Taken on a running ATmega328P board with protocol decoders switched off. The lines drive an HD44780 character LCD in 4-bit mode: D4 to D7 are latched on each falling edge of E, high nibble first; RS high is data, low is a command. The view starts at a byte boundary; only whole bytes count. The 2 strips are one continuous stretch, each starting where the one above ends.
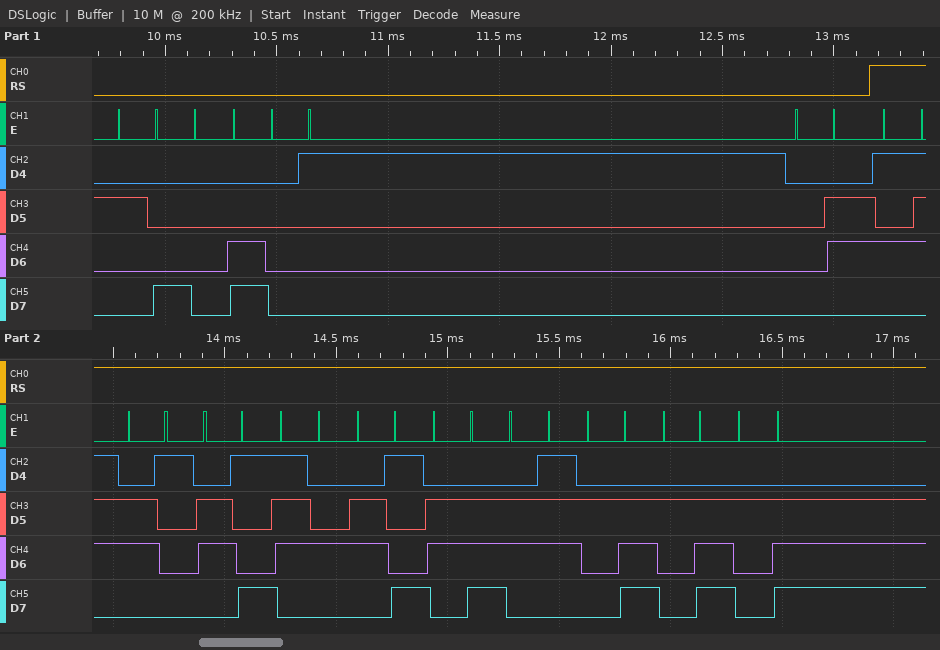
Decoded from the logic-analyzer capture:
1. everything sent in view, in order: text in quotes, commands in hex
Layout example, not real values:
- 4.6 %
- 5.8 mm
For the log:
- 0x28 0x0C 0x01 0x06 "Waiting..."
